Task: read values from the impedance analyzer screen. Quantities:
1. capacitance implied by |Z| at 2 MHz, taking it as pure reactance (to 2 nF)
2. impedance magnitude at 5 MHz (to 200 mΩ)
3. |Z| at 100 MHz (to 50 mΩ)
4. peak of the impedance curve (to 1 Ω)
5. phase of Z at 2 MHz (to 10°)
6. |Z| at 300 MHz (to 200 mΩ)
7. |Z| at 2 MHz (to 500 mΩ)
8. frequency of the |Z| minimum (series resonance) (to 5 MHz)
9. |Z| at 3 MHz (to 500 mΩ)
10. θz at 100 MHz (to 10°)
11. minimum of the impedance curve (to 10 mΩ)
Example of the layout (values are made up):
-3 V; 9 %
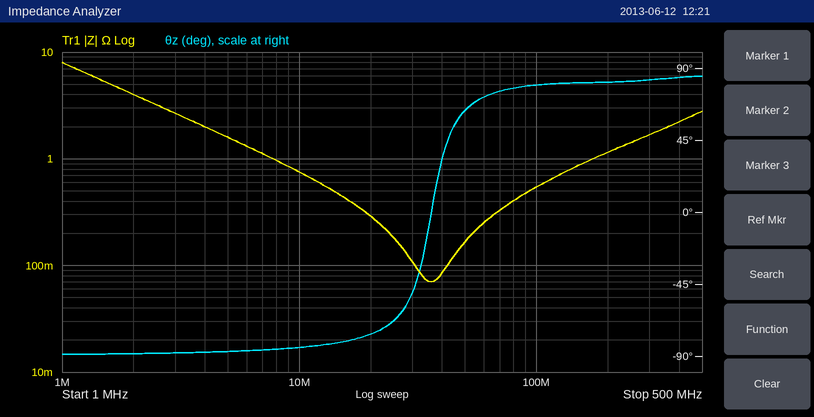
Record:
20 nF; 1.6 Ω; 550 mΩ; 8 Ω; -90°; 1.6 Ω; 4.0 Ω; 35 MHz; 2.5 Ω; 80°; 70 mΩ
